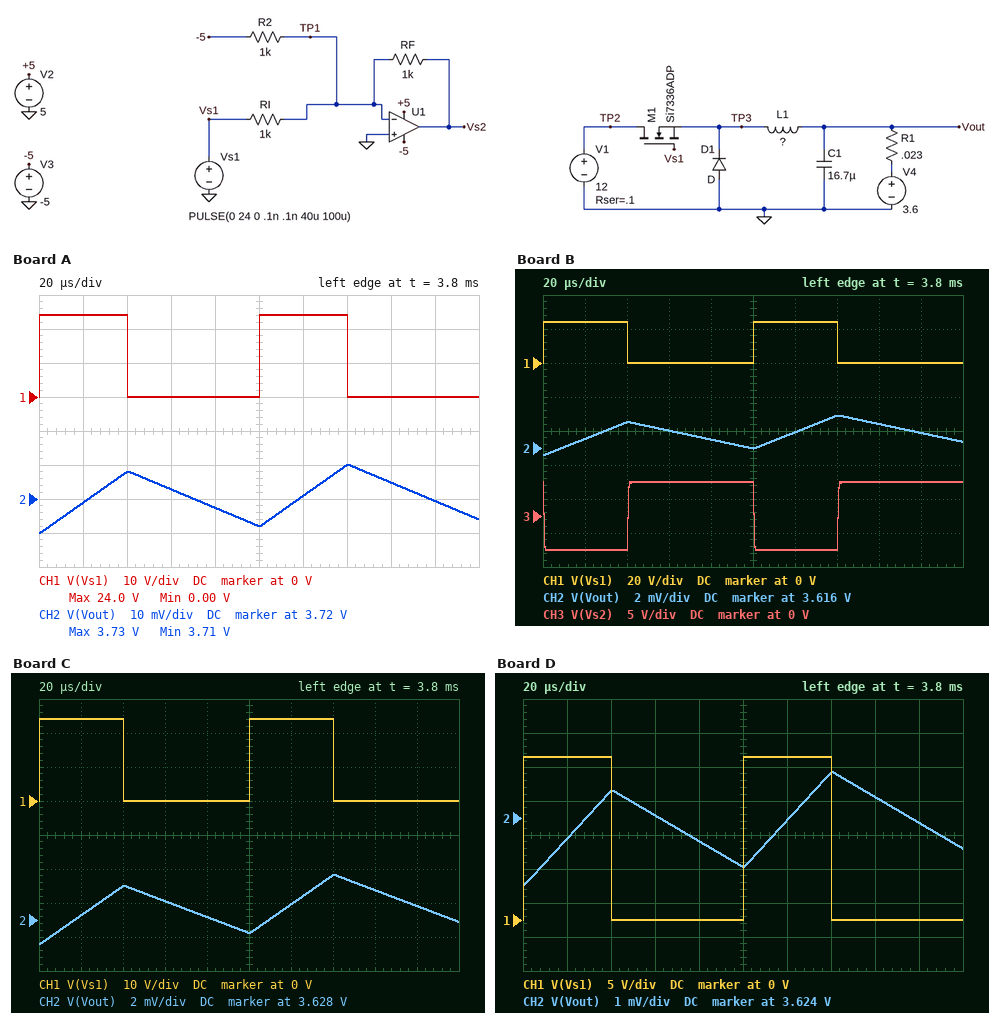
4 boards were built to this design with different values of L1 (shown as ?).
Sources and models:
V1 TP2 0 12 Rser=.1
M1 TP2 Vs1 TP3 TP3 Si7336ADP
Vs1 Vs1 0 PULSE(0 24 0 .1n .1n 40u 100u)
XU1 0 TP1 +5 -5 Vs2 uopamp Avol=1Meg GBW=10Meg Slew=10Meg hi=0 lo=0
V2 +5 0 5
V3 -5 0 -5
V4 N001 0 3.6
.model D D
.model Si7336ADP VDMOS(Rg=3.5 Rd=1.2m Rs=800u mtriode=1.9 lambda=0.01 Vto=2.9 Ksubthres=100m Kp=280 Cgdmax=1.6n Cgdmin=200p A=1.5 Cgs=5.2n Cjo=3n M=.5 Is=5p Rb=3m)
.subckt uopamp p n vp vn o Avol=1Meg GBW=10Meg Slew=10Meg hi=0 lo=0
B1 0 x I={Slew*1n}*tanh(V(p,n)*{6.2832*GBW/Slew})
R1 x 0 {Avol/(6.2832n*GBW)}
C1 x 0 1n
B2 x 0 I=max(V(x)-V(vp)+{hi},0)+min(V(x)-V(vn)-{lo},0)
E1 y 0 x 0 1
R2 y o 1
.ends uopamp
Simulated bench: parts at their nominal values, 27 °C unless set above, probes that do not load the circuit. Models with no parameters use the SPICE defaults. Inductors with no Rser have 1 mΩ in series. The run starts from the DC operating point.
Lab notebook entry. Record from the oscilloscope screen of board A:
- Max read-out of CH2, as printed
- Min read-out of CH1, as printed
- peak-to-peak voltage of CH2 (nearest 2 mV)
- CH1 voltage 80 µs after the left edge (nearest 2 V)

3.73 V
0.00 V
20 mV
0 V
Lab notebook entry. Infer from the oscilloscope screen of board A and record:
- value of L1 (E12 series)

390 µH
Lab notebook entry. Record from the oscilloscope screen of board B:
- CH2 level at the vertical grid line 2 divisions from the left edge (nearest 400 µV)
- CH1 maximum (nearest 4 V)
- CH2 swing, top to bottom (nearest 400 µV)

3.6176 V
24 V
2.4 mV
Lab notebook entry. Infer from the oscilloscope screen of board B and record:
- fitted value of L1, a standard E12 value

3.9 mH
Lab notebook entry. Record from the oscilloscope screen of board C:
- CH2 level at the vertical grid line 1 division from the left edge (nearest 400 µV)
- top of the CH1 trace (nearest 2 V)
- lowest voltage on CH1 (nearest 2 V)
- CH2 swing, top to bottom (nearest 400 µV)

3.6284 V
24 V
0 V
4.0 mV
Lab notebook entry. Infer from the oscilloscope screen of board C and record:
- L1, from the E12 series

2.2 mH
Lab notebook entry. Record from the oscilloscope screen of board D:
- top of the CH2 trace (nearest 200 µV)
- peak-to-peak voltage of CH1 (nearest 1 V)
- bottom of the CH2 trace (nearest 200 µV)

3.6254 V
24 V
3.6220 V
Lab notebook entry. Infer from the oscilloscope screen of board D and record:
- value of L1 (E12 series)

2.7 mH
